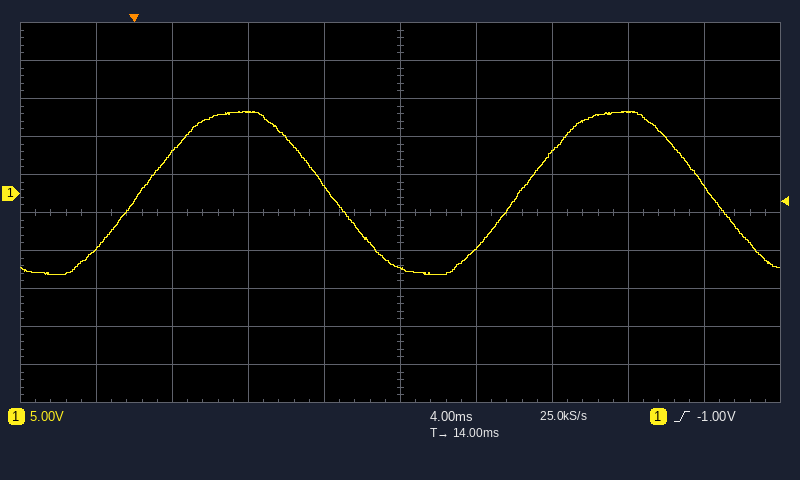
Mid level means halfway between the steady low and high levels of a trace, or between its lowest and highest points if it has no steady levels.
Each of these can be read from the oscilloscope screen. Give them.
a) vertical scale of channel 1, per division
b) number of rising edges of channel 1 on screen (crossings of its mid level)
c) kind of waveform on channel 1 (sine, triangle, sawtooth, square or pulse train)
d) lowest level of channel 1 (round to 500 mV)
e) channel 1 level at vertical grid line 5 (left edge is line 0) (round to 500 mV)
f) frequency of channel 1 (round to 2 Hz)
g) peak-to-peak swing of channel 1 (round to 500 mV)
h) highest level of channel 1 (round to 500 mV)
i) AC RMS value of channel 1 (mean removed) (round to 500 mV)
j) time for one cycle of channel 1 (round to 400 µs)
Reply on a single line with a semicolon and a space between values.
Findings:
5 V; 2; sine; -10.5 V; -10.0 V; 50 Hz; 21.5 V; 11.0 V; 7.5 V; 20.0 ms
